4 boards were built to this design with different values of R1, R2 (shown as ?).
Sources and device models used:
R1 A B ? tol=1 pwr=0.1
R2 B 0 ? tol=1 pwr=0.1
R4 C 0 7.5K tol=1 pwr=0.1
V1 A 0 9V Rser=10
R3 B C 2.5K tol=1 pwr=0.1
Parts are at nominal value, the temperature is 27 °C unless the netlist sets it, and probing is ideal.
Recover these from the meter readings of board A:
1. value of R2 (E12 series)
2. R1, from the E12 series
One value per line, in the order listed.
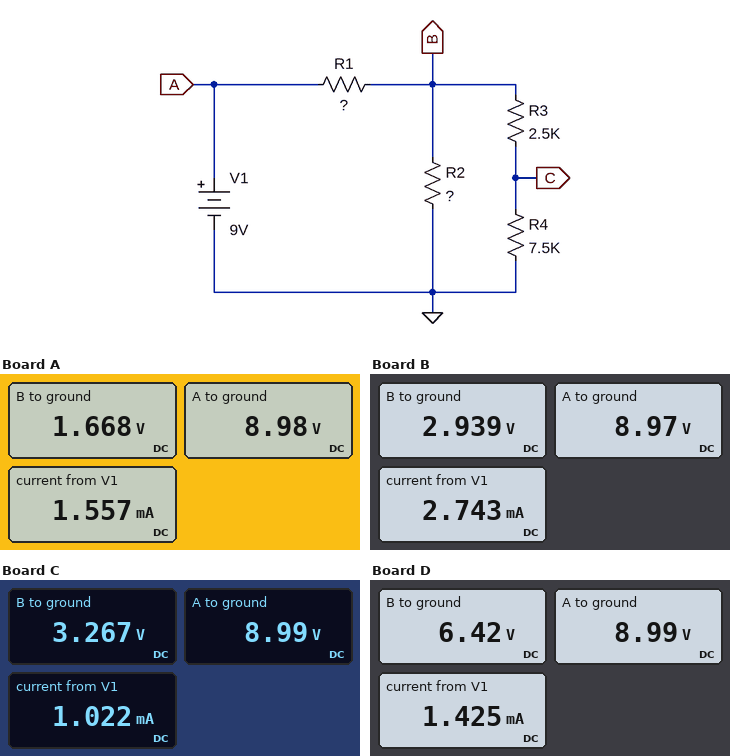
1.2 kΩ
4.7 kΩ
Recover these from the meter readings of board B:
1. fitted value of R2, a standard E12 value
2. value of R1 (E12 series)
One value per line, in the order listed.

1.2 kΩ
2.2 kΩ
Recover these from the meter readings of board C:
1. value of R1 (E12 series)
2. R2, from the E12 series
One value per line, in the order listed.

5.6 kΩ
4.7 kΩ
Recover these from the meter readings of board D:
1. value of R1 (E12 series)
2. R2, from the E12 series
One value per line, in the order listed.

1.8 kΩ
8.2 kΩ
